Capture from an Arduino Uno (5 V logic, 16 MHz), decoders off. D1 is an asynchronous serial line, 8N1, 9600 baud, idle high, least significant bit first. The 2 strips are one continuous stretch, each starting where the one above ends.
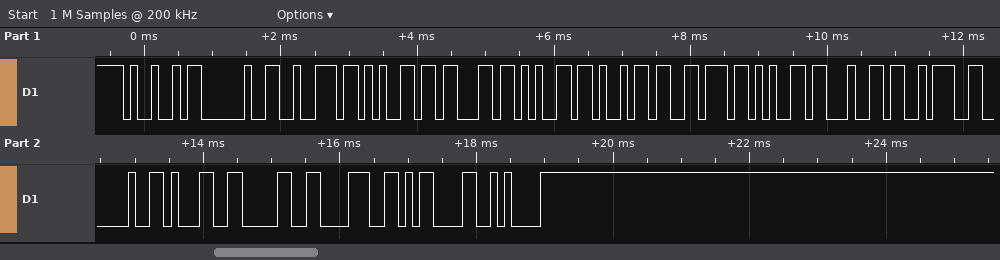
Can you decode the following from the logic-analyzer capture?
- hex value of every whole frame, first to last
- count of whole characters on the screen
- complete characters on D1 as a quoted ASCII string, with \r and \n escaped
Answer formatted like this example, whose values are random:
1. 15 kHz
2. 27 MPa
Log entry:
1. 49 20 72 65 63 65 69 76 65 64 3A 20 31 30 38 0D 0A
2. 17
3. "I received: 108\r\n"
